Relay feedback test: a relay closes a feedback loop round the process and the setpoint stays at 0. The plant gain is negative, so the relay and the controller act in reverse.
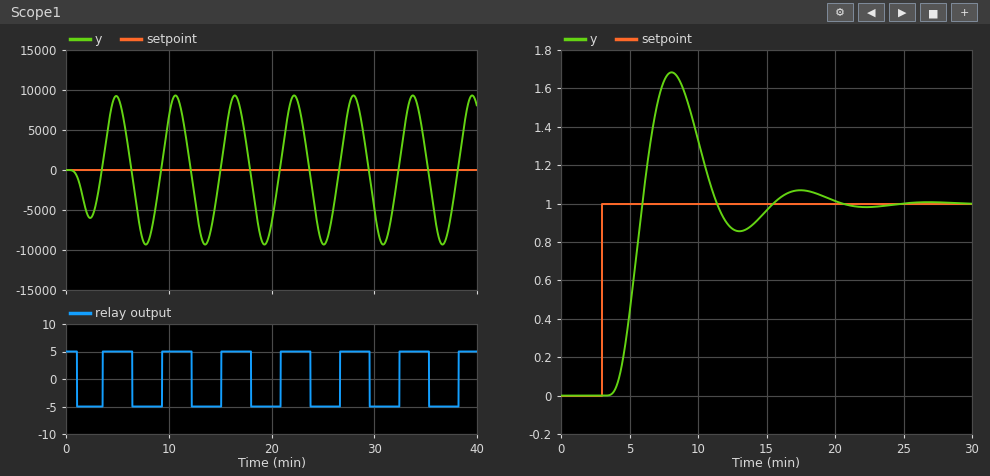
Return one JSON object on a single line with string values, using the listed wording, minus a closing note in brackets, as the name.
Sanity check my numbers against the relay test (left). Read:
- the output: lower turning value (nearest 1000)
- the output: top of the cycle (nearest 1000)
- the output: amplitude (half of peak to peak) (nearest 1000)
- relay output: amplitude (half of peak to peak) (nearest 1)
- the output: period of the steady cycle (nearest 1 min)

{"the output: lower turning value": "-9000", "the output: top of the cycle": "9000", "the output: amplitude (half of peak to peak)": "9000", "relay output: amplitude (half of peak to peak)": "5", "the output: period of the steady cycle": "6 min"}
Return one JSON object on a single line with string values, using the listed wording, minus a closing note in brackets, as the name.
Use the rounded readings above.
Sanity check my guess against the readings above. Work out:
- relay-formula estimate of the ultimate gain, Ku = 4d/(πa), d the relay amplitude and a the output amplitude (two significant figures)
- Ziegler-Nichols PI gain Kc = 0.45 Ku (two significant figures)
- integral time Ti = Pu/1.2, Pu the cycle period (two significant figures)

{"relay-formula estimate of the ultimate gain, Ku = 4d/(πa), d the relay amplitude and a the output amplitude": "0.00071", "Ziegler-Nichols PI gain Kc = 0.45 Ku": "0.00032", "integral time Ti = Pu/1.2, Pu the cycle period": "5.0 min"}
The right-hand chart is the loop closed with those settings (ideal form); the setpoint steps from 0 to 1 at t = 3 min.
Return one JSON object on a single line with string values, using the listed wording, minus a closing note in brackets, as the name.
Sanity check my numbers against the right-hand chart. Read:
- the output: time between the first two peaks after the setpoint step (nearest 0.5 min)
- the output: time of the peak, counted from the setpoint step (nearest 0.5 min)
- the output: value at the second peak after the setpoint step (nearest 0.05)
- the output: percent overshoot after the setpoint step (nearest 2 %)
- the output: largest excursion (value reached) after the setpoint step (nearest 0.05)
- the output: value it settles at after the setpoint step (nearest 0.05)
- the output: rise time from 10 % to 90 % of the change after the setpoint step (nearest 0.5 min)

{"the output: time between the first two peaks after the setpoint step": "9.5 min", "the output: time of the peak, counted from the setpoint step": "5.0 min", "the output: value at the second peak after the setpoint step": "1.05", "the output: percent overshoot after the setpoint step": "68 %", "the output: largest excursion (value reached) after the setpoint step": "1.70", "the output: value it settles at after the setpoint step": "1.00", "the output: rise time from 10 % to 90 % of the change after the setpoint step": "1.5 min"}
